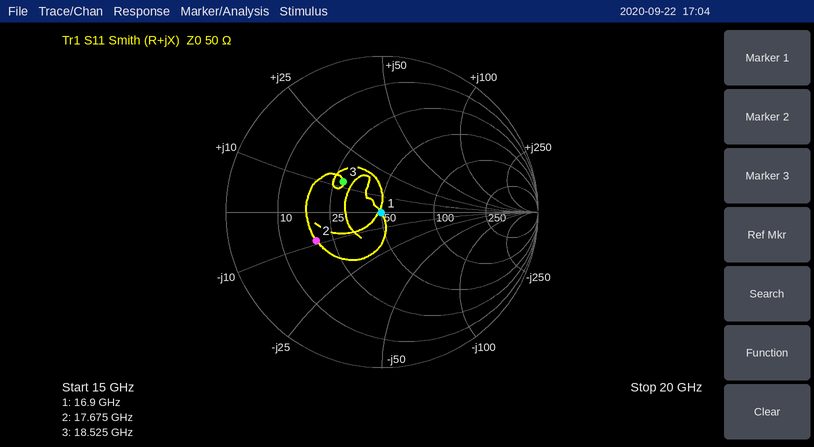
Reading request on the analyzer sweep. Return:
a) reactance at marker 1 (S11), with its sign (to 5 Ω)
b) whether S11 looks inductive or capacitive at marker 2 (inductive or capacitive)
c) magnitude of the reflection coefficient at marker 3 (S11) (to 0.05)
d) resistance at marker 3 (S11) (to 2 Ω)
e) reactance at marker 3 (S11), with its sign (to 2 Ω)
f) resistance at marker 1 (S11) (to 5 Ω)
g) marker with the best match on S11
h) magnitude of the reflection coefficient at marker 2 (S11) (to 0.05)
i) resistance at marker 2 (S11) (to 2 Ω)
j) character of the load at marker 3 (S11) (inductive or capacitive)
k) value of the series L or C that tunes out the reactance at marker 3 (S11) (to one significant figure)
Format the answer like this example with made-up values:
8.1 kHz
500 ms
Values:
0 Ω
capacitive
0.30
28 Ω
+12 Ω
50 Ω
marker 1
0.45
20 Ω
inductive
700 fF
